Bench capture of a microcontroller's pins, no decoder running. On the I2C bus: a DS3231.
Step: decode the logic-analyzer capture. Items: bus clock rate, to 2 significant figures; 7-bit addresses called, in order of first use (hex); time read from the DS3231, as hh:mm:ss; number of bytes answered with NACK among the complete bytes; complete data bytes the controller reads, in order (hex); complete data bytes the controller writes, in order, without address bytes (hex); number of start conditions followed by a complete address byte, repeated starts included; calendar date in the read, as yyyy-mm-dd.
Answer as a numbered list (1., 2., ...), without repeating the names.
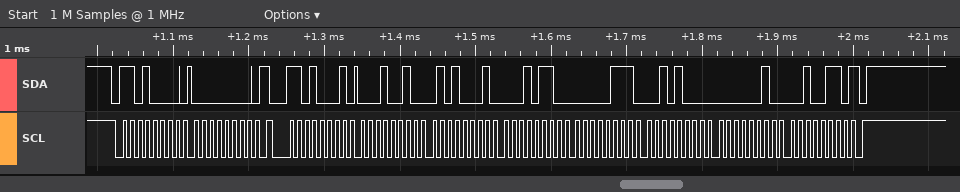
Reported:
1. 100 kHz
2. 0x68
3. 16:51:12
4. 1
5. 12 51 16 07 28 02 26
6. 00
7. 2
8. 2026-02-28
